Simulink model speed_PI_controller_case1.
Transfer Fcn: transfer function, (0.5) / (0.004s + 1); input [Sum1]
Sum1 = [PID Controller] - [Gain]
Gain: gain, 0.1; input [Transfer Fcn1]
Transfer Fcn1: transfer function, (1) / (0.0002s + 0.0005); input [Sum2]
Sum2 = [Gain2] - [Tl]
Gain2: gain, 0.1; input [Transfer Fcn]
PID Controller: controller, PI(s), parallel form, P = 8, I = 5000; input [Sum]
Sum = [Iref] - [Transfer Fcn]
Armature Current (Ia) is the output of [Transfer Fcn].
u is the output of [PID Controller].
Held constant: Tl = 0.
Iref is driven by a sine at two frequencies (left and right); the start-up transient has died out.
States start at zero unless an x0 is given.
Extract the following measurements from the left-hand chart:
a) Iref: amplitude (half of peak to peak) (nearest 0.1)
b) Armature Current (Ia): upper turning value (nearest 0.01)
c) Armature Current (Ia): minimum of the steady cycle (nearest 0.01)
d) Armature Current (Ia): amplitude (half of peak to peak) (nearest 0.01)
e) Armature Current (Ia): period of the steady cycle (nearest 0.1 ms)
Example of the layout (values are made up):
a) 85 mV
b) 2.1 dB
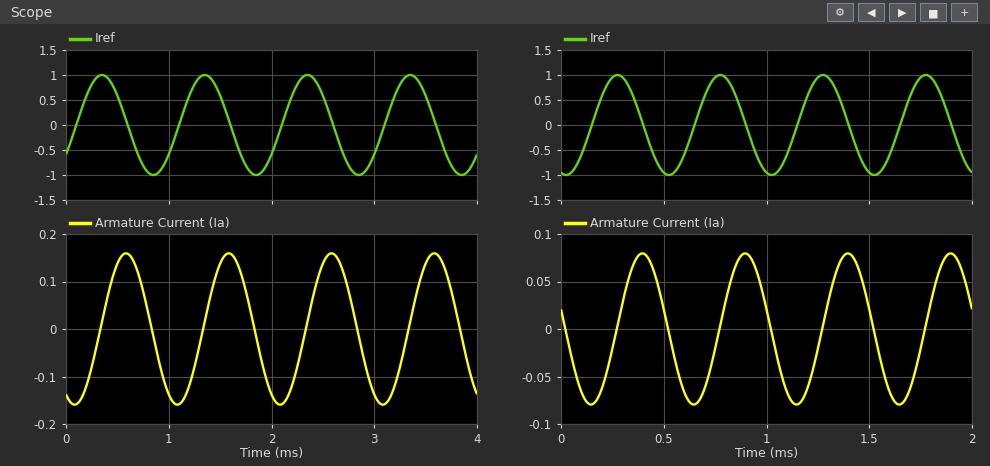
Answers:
a) 1.0
b) 0.16
c) -0.16
d) 0.16
e) 1.0 ms
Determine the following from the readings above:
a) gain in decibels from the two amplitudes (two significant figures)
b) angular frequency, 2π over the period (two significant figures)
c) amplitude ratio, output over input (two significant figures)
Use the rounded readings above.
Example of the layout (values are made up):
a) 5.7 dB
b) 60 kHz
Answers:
a) -16 dB
b) 6.3 rad/ms
c) 0.16
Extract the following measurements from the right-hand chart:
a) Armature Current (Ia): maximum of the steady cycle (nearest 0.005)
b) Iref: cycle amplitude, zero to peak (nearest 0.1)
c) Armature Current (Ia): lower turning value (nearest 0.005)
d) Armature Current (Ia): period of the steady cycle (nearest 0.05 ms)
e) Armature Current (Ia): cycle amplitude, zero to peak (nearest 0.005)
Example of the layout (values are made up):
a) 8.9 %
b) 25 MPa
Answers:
a) 0.080
b) 1.0
c) -0.080
d) 0.50 ms
e) 0.080
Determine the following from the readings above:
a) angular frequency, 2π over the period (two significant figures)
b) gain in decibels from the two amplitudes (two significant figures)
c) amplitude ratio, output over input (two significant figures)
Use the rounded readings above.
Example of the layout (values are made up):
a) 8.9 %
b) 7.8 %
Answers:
a) 13 rad/ms
b) -22 dB
c) 0.080
